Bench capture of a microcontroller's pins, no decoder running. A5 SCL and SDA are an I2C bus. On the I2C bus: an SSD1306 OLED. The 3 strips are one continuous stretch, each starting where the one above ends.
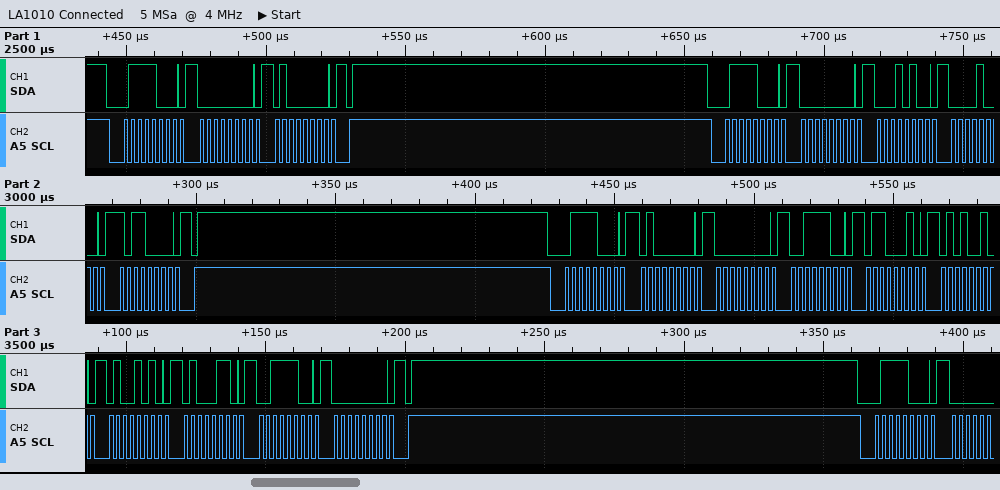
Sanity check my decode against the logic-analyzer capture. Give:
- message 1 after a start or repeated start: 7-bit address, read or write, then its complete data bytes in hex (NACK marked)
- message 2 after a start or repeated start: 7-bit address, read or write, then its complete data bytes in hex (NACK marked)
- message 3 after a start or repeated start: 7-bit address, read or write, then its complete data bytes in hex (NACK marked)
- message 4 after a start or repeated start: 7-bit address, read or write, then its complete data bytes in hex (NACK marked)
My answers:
0x3C write: 00 40
0x3C write: 00 14 08 B0
0x3C write: 40 00 3C 62 52 4A 46 3C 00
0x3C write
